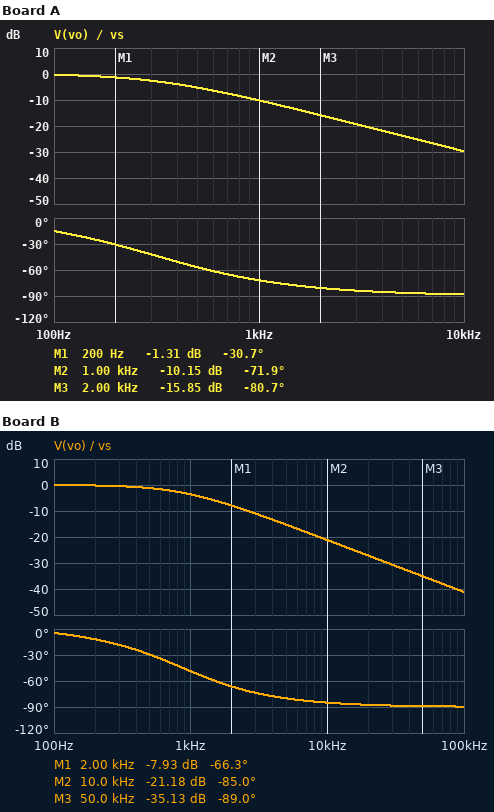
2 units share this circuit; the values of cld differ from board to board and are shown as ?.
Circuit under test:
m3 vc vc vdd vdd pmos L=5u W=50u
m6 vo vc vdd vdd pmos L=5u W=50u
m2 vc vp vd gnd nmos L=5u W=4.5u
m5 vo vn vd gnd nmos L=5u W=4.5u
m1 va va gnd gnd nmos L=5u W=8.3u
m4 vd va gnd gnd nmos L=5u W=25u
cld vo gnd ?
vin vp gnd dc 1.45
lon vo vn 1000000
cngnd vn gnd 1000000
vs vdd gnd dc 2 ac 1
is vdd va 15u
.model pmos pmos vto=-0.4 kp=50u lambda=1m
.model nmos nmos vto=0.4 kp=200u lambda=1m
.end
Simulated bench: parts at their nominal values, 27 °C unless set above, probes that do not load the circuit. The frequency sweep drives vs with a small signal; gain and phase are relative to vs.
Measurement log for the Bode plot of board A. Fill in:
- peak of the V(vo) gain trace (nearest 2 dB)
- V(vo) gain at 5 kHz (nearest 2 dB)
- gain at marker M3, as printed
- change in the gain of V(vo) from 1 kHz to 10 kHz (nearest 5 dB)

0 dB
-24 dB
-15.85 dB
-20 dB
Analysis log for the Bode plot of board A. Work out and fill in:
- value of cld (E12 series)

22 pF
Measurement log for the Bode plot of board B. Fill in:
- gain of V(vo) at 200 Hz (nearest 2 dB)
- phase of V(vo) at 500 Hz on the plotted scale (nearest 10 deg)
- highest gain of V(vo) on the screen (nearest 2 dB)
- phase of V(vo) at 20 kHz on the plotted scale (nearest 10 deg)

0 dB
-30 deg
0 dB
-90 deg
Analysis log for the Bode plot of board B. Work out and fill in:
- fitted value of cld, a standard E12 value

8.2 pF
